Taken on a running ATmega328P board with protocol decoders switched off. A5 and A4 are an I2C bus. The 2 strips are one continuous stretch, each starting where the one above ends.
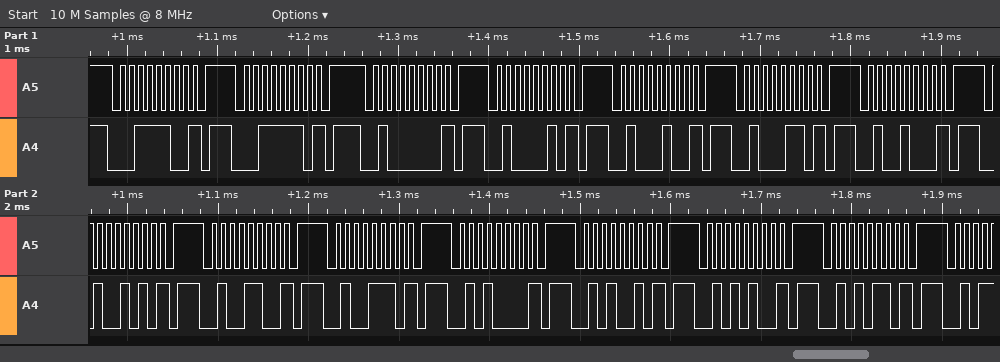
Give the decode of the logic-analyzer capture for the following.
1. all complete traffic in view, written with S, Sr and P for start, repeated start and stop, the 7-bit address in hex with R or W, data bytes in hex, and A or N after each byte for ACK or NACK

S 1EW N P S 1FW N P S 20W N P S 21W N P S 22W N P S 23W N P S 24W N P S 25W N P S 26W N P S 27W N P S 28W N P S 29W N P S 2AW N P S 2BW N P
